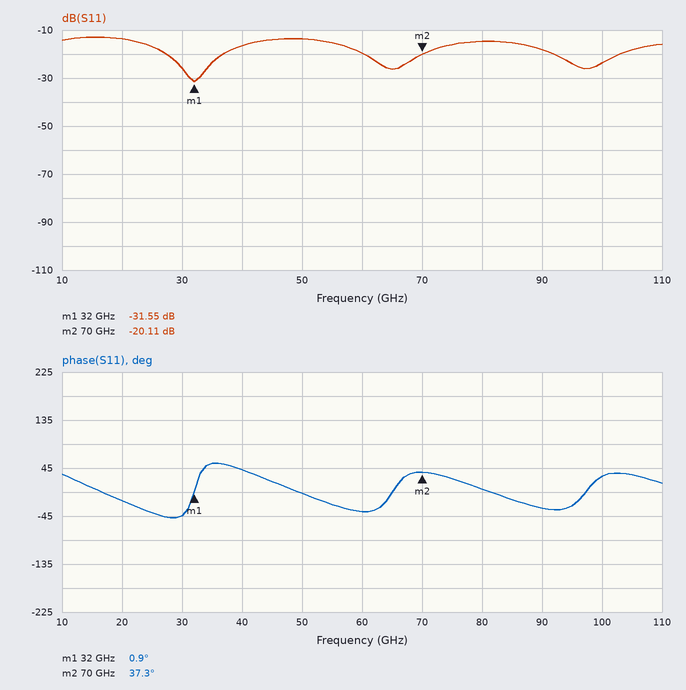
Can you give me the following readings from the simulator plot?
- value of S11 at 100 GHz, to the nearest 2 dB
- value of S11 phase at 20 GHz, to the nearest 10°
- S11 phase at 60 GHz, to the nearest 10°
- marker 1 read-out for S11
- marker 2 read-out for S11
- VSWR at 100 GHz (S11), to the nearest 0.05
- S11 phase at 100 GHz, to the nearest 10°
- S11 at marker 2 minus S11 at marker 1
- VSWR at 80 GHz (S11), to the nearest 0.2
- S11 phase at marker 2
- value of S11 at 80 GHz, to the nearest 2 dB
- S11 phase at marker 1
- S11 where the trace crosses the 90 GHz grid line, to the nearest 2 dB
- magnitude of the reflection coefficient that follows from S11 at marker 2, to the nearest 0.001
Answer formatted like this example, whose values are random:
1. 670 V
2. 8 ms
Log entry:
1. -24 dB
2. -20°
3. -40°
4. -31.55 dB
5. -20.11 dB
6. 1.15
7. 30°
8. 11.44 dB
9. 1.4
10. 37.3°
11. -14 dB
12. 0.9°
13. -18 dB
14. 0.099
